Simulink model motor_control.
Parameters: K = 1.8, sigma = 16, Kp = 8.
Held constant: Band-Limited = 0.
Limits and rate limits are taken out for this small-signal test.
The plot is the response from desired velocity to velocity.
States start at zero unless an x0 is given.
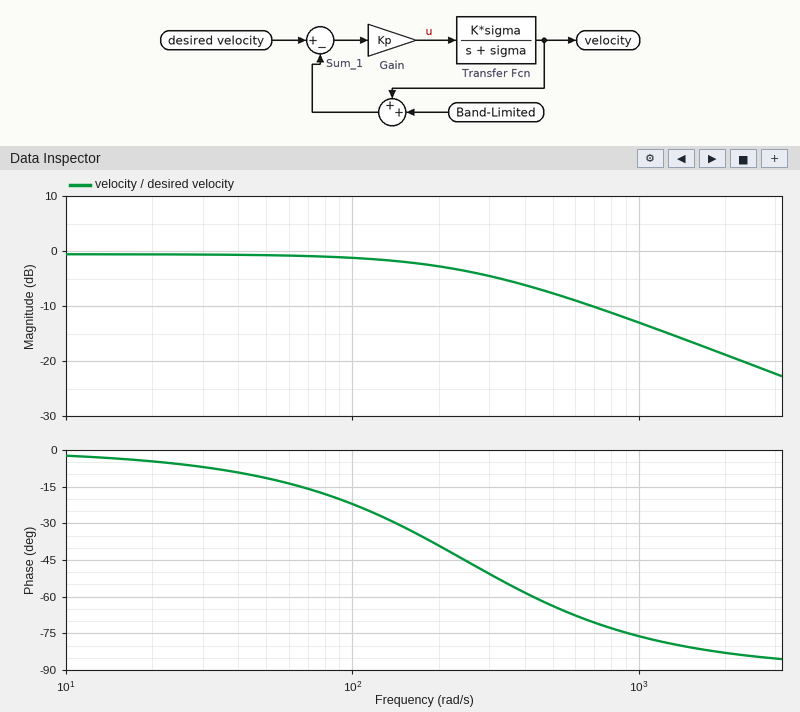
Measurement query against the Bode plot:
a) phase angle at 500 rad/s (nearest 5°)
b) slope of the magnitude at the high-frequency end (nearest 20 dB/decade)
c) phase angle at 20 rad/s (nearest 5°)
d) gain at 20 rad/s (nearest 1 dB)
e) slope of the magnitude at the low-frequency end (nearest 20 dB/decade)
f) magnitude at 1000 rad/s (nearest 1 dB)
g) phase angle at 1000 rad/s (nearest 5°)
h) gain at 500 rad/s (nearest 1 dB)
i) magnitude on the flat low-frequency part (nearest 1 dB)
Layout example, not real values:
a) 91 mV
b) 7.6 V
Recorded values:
a) -65°
b) -20 dB/decade
c) -5°
d) -1 dB
e) 0 dB/decade
f) -13 dB
g) -75°
h) -8 dB
i) -1 dB
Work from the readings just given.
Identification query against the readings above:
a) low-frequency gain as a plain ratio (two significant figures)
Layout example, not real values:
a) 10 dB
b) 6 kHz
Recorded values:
a) 0.89
